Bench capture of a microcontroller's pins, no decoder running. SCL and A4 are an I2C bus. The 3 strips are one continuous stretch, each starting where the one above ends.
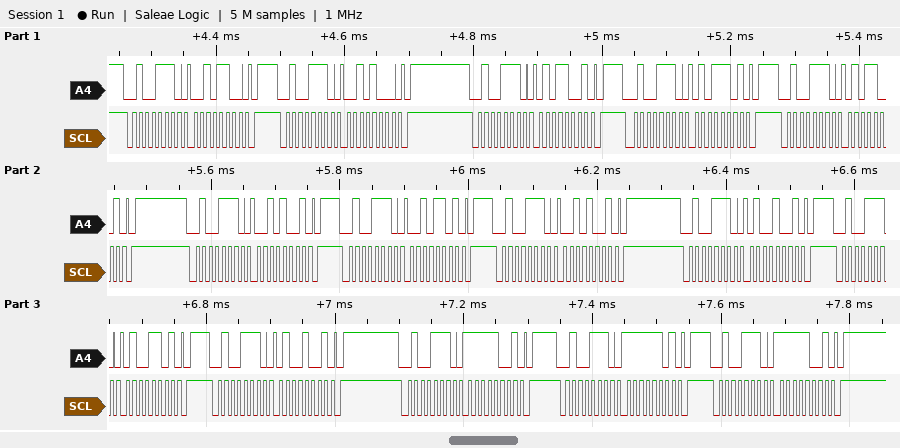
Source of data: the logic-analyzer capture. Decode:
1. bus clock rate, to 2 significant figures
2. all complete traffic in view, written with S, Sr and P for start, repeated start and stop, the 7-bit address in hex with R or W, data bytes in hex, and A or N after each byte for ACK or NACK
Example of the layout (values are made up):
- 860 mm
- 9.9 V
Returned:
- 100 kHz
- S 27W A 2C A P S 27W A 28 A P S 27W A 59 A P S 27W A 5D A P S 27W A 59 A P S 27W A 29 A P S 27W A 2D A P S 27W A 29 A P S 27W A 49 A P S 27W A 4D A P S 27W A 49 A P S 27W A F9 A P S 27W A FD A P S 27W A F9 A P
